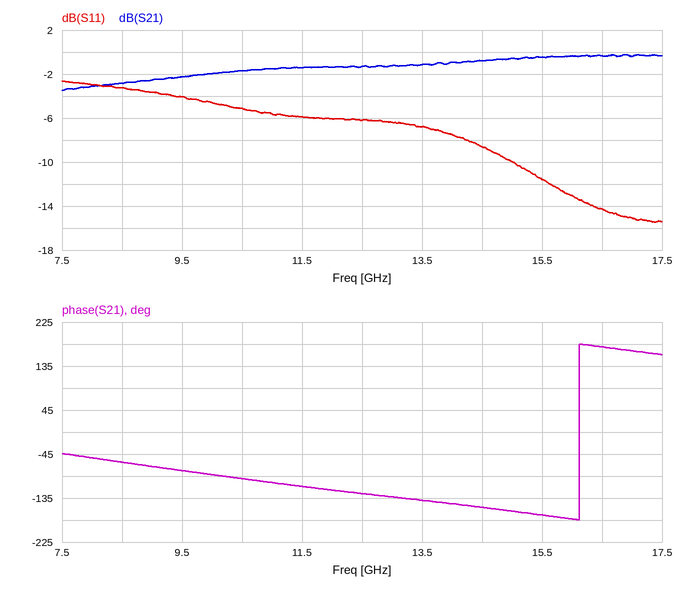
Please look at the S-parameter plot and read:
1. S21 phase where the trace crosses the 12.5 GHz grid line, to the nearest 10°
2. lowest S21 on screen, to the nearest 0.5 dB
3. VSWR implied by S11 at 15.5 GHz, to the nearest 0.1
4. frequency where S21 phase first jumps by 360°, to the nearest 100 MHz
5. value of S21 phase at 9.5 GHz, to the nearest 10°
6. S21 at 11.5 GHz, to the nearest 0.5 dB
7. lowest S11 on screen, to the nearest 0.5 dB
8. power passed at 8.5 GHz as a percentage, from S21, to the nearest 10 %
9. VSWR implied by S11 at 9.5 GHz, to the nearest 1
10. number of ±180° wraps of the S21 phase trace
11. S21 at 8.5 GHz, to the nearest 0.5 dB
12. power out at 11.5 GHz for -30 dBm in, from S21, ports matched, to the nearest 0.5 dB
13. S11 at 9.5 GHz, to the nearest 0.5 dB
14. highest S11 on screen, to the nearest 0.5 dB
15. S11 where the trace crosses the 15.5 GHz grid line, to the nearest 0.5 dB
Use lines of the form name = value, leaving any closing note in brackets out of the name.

S21 phase where the trace crosses the 12.5 GHz grid line, to the nearest 10° = -130°
lowest S21 on screen, to the nearest 0.5 dB = -3.5 dB
VSWR implied by S11 at 15.5 GHz, to the nearest 0.1 = 1.7
frequency where S21 phase first jumps by 360°, to the nearest 100 MHz = 16.1 GHz
value of S21 phase at 9.5 GHz, to the nearest 10° = -80°
S21 at 11.5 GHz, to the nearest 0.5 dB = -1.5 dB
lowest S11 on screen, to the nearest 0.5 dB = -15.5 dB
power passed at 8.5 GHz as a percentage, from S21, to the nearest 10 % = 50 %
VSWR implied by S11 at 9.5 GHz, to the nearest 1 = 4
number of ±180° wraps of the S21 phase trace = 1
S21 at 8.5 GHz, to the nearest 0.5 dB = -3.0 dB
power out at 11.5 GHz for -30 dBm in, from S21, ports matched, to the nearest 0.5 dB = -31.5 dBm
S11 at 9.5 GHz, to the nearest 0.5 dB = -4.0 dB
highest S11 on screen, to the nearest 0.5 dB = -2.5 dB
S11 where the trace crosses the 15.5 GHz grid line, to the nearest 0.5 dB = -11.5 dB
